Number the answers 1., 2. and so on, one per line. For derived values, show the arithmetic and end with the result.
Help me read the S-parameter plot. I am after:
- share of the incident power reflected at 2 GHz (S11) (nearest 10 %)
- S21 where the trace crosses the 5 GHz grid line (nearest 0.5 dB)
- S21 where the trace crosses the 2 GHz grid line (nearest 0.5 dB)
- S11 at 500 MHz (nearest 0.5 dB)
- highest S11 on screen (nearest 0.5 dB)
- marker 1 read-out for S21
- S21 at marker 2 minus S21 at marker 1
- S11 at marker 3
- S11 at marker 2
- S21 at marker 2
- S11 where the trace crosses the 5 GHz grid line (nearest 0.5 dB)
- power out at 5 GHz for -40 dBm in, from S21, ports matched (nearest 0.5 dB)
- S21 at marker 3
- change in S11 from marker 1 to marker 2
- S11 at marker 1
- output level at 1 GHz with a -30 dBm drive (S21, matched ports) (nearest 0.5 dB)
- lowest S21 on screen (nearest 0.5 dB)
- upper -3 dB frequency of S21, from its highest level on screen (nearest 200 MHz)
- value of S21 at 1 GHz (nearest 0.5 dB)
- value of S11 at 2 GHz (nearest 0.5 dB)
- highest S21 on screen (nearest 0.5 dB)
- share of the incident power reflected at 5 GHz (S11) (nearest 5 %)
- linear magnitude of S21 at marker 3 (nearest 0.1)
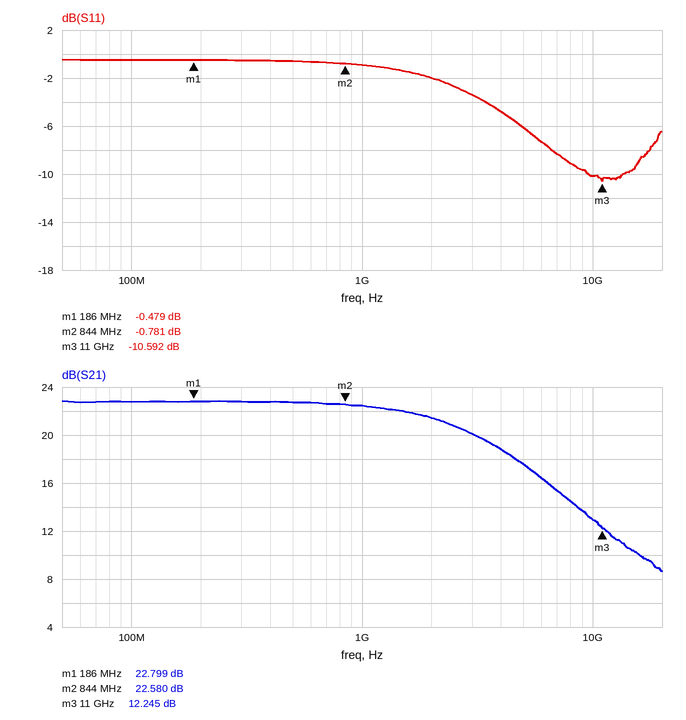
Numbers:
1. 10^(-2/10) ≈ 63.1 %, so 60 % to the nearest 10 %
2. 17.5 dB
3. 21.5 dB
4. -0.5 dB
5. -0.5 dB
6. 22.799 dB
7. 22.58 − (22.799) = -0.219 dB
8. -10.592 dB
9. -0.781 dB
10. 22.580 dB
11. -6.0 dB
12. -40 dBm + (17.5 dB) = -22.5 dBm
13. 12.245 dB
14. -0.781 − (-0.479) = -0.302 dB
15. -0.479 dB
16. -30 dBm + (22.5 dB) = -7.5 dBm
17. 8.5 dB
18. 3.2 GHz
19. 22.5 dB
20. -2.0 dB
21. 23.0 dB
22. 10^(-6/10) ≈ 25 %
23. 10^(12.245/20) ≈ 4.1
